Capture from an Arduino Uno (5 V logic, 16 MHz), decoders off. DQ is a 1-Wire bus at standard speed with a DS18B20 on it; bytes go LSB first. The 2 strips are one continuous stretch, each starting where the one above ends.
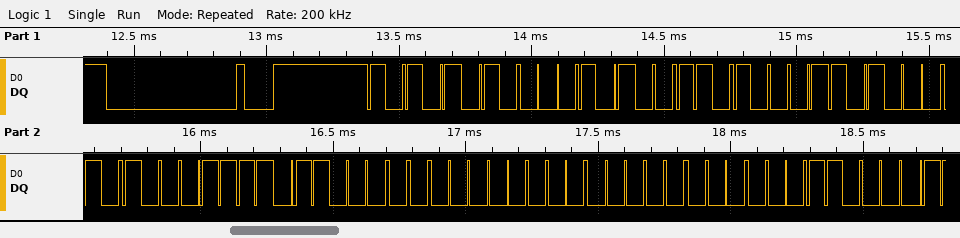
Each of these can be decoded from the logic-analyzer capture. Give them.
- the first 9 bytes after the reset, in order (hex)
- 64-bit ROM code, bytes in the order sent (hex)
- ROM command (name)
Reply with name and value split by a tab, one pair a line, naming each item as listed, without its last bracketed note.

the first 9 bytes after the reset, in order	55 28 8B 45 F1 06 00 00 18
64-bit ROM code, bytes in the order sent	28 8B 45 F1 06 00 00 18
ROM command	Match ROM
